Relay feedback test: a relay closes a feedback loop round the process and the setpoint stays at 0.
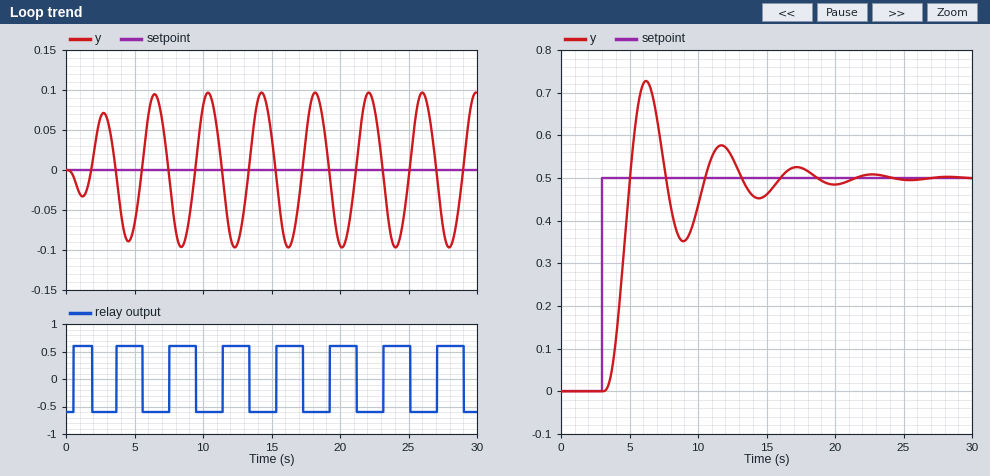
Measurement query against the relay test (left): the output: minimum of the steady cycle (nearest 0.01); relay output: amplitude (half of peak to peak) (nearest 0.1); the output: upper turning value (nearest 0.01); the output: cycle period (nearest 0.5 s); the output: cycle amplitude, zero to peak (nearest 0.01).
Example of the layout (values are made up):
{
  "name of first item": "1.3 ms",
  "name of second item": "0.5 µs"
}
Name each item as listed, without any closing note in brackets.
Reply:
{
  "the output: minimum of the steady cycle": "-0.10",
  "relay output: amplitude (half of peak to peak)": "0.6",
  "the output: upper turning value": "0.10",
  "the output: cycle period": "4.0 s",
  "the output: cycle amplitude, zero to peak": "0.10"
}
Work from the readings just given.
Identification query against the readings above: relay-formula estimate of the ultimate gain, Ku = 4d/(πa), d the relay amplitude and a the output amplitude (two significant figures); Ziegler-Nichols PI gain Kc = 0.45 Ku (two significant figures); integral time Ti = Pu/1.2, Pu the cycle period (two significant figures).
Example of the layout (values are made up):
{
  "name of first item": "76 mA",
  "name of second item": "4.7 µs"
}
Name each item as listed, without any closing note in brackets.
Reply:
{
  "relay-formula estimate of the ultimate gain, Ku = 4d/(πa), d the relay amplitude and a the output amplitude": "7.6",
  "Ziegler-Nichols PI gain Kc = 0.45 Ku": "3.4",
  "integral time Ti = Pu/1.2, Pu the cycle period": "3.3 s"
}
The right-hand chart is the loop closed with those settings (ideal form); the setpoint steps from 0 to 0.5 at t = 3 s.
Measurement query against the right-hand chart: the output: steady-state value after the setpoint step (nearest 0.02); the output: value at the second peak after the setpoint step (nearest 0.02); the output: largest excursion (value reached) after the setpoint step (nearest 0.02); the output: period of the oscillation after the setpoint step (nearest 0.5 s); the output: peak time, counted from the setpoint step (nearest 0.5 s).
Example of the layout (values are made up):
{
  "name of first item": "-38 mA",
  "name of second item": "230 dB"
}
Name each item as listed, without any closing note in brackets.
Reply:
{
  "the output: steady-state value after the setpoint step": "0.50",
  "the output: value at the second peak after the setpoint step": "0.58",
  "the output: largest excursion (value reached) after the setpoint step": "0.72",
  "the output: period of the oscillation after the setpoint step": "5.5 s",
  "the output: peak time, counted from the setpoint step": "3.0 s"
}
